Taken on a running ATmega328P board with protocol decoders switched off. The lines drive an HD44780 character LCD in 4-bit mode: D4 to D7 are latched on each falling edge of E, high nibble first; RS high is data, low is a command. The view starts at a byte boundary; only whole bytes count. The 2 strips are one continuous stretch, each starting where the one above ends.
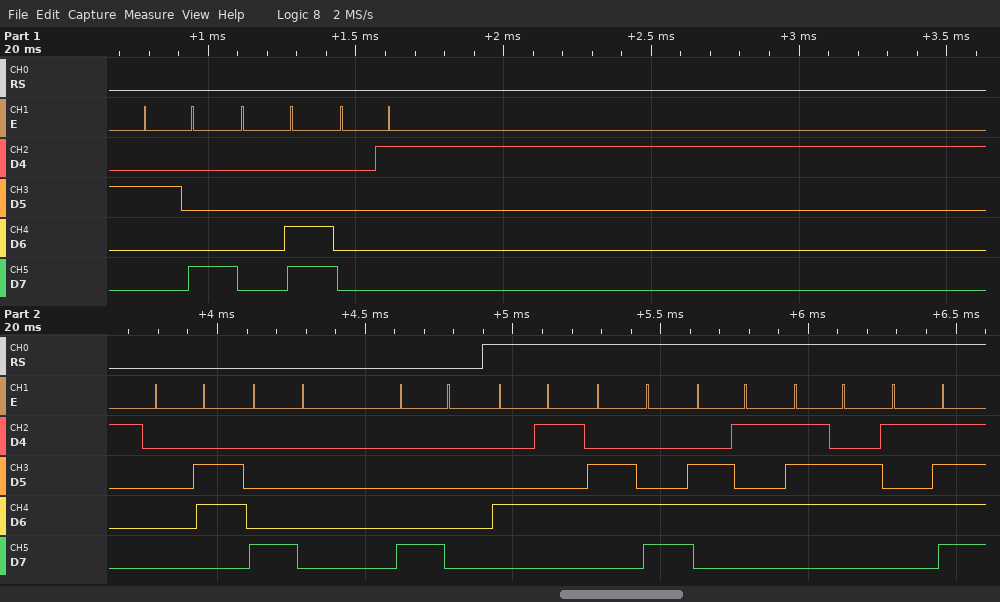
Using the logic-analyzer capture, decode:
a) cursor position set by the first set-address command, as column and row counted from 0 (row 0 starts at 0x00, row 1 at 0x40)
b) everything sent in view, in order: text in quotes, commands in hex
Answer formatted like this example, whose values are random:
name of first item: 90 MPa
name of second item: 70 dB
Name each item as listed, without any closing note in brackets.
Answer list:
cursor position set by the first set-address command, as column and row counted from 0: column 0, row 0
everything sent in view, in order: text in quotes, commands in hex: 0x28 0x0C 0x01 0x06 0x80 0x80 "Elev_"
